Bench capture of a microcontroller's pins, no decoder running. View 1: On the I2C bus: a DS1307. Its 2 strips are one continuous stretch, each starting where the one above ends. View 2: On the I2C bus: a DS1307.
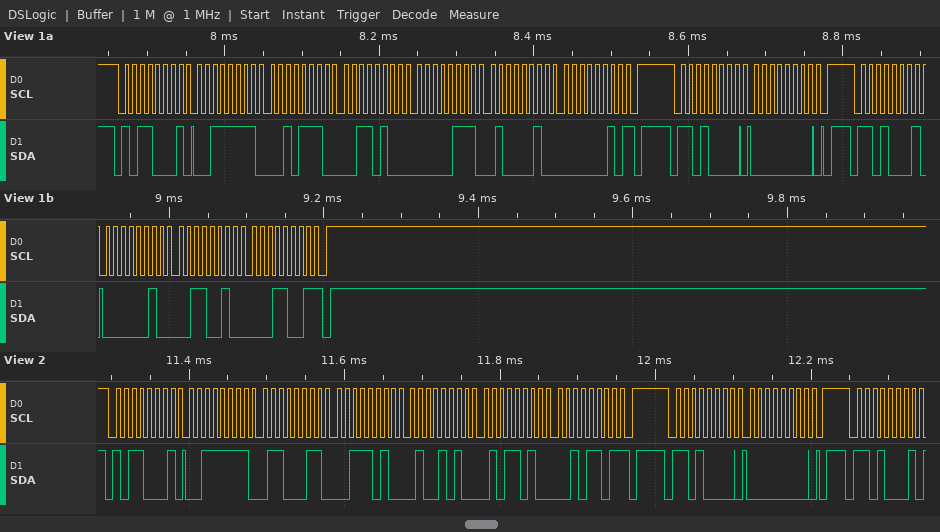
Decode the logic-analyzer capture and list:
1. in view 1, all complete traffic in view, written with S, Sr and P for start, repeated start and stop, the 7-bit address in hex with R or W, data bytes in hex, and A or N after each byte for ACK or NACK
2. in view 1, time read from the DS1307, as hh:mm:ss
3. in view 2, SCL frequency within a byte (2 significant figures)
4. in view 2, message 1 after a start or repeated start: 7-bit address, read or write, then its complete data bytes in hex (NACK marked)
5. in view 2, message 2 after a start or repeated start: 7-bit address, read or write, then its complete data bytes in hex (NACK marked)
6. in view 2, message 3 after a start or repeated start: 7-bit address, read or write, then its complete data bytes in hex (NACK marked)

S 58R A 3F A 2E A 34 A 07 A 42 A 02 N P S 68W A 00 A P S 68R A 02 A 32 A 19 N P
19:32:02
100 kHz
0x58 read: 3F 63 3A 4A 5A 2D NACK
0x68 write: 00
0x68 read
